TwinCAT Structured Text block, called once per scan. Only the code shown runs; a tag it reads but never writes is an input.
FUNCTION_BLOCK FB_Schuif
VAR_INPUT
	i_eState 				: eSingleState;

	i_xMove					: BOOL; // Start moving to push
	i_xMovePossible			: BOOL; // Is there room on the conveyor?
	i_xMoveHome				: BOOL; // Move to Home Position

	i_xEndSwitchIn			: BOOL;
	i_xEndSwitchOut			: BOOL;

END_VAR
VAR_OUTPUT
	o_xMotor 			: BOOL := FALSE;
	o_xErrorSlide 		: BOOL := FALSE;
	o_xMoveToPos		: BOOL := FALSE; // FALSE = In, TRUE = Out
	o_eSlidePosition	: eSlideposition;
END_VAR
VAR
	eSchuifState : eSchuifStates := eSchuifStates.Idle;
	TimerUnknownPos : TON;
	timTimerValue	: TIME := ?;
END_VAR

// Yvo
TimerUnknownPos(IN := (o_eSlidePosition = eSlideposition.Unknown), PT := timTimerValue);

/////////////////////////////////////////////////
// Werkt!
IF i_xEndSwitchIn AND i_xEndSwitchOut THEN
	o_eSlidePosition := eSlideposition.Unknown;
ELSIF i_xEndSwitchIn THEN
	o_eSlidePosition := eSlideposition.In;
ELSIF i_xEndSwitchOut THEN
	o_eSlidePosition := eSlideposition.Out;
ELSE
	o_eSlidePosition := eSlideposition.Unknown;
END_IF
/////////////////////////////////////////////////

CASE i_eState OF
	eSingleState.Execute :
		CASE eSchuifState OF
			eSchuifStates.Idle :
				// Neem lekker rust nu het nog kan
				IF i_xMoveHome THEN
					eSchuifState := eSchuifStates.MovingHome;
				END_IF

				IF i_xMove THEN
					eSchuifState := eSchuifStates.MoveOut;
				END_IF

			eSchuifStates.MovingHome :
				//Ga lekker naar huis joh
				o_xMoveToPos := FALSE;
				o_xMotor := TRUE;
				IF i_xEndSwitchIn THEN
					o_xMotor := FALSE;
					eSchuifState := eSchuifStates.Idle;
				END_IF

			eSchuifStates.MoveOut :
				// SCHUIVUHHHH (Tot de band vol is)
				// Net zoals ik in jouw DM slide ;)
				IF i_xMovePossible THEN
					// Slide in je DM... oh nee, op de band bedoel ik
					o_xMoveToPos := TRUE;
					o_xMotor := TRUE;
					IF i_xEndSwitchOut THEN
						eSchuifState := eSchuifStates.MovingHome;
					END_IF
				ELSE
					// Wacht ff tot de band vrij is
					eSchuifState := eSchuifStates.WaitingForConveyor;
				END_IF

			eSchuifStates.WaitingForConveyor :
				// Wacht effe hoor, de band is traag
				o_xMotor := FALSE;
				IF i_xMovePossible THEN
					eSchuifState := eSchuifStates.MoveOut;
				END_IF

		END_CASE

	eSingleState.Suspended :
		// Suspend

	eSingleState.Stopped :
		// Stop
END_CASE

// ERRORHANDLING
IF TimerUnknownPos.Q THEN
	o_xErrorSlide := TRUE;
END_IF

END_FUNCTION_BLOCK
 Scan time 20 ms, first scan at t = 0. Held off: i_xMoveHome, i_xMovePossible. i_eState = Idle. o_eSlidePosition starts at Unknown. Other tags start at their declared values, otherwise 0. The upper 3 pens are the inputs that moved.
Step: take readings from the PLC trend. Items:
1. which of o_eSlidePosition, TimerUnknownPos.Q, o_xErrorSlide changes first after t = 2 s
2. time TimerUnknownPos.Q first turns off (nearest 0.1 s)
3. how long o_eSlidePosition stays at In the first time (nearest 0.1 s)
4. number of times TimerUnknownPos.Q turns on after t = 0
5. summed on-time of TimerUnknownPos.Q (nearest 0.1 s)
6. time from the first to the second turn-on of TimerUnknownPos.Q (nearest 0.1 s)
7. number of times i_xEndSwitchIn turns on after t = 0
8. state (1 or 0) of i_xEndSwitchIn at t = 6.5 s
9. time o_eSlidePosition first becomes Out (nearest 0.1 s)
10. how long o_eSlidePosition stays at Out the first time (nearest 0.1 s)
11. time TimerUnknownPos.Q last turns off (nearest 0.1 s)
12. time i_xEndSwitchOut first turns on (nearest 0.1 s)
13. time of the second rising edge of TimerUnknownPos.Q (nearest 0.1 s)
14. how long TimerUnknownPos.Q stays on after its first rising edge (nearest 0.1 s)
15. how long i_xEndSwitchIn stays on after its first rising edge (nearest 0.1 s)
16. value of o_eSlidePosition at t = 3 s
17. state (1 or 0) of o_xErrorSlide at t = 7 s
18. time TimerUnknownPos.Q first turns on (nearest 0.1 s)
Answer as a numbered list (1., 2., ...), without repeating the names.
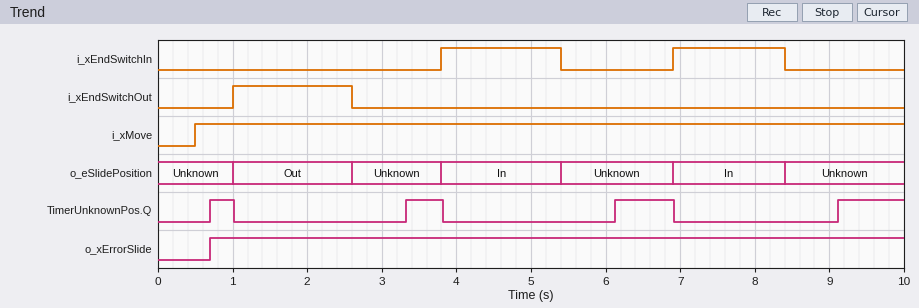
1. o_eSlidePosition
2. 1.0 s
3. 1.6 s
4. 4
5. 2.5 s
6. 2.6 s
7. 2
8. 0
9. 1.0 s
10. 1.6 s
11. 6.9 s
12. 1.0 s
13. 3.3 s
14. 0.3 s
15. 1.6 s
16. Unknown
17. 1
18. 0.7 s
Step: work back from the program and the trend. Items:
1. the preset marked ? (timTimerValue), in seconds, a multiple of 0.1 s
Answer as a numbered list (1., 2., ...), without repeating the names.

1. 0.7 s
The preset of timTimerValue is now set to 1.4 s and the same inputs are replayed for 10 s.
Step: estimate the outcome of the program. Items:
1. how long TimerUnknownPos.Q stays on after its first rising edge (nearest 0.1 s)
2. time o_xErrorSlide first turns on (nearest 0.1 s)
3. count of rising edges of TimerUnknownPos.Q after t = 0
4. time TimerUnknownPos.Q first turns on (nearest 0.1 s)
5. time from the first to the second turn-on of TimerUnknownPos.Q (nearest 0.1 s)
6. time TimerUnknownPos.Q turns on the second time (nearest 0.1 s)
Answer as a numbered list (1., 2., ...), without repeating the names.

1. 0.1 s
2. 6.8 s
3. 2
4. 6.8 s
5. 3.0 s
6. 9.8 s
